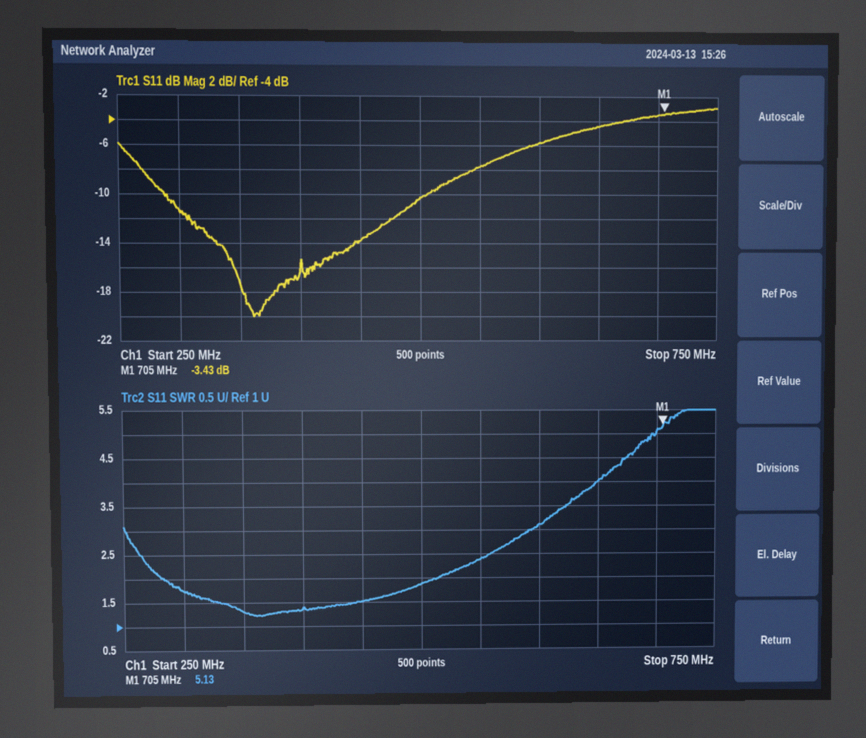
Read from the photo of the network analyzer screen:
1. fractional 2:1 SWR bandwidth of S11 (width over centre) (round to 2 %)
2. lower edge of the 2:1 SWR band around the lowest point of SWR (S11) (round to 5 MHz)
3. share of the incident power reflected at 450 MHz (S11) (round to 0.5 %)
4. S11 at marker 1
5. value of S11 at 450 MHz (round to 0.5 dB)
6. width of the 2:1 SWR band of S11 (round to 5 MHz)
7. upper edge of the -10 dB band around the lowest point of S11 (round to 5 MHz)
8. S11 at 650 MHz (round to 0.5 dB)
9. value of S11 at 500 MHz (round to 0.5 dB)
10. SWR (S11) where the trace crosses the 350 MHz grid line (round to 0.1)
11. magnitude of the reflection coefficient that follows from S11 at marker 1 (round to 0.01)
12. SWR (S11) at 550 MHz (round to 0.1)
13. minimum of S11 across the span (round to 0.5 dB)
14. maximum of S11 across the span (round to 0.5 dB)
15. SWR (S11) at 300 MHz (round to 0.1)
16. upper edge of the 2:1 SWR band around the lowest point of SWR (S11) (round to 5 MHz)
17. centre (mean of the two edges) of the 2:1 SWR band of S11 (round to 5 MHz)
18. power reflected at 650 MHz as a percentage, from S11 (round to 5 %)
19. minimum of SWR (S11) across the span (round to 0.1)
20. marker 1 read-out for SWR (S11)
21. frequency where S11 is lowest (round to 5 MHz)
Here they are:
58 %
285 MHz
4.0 %
-3.43 dB
-14.0 dB
230 MHz
505 MHz
-4.5 dB
-10.5 dB
1.3
0.67
2.4
-20.0 dB
-3.0 dB
1.7
515 MHz
400 MHz
35 %
1.2
5.13
360 MHz
